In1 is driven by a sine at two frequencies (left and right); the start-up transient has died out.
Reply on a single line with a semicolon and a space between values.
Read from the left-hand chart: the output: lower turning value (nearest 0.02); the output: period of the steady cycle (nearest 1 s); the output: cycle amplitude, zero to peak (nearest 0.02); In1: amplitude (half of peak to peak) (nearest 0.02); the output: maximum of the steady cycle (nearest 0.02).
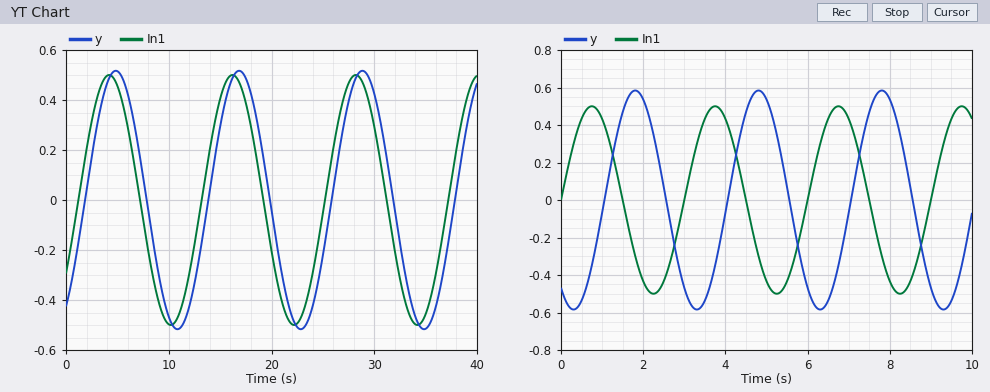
-0.52; 12 s; 0.52; 0.50; 0.52
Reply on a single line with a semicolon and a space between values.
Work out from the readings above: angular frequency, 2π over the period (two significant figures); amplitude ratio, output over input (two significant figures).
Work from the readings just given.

0.52 rad/s; 1.0
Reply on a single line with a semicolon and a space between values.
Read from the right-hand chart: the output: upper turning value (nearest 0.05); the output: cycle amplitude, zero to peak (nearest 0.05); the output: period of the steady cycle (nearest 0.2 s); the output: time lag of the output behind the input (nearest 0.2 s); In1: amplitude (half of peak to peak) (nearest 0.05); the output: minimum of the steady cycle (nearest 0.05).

0.60; 0.60; 3.0 s; 1.0 s; 0.50; -0.60
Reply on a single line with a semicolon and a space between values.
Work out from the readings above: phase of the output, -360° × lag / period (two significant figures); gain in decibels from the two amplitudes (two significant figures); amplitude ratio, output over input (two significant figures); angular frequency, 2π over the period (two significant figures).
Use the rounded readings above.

-120°; 1.6 dB; 1.2; 2.1 rad/s
